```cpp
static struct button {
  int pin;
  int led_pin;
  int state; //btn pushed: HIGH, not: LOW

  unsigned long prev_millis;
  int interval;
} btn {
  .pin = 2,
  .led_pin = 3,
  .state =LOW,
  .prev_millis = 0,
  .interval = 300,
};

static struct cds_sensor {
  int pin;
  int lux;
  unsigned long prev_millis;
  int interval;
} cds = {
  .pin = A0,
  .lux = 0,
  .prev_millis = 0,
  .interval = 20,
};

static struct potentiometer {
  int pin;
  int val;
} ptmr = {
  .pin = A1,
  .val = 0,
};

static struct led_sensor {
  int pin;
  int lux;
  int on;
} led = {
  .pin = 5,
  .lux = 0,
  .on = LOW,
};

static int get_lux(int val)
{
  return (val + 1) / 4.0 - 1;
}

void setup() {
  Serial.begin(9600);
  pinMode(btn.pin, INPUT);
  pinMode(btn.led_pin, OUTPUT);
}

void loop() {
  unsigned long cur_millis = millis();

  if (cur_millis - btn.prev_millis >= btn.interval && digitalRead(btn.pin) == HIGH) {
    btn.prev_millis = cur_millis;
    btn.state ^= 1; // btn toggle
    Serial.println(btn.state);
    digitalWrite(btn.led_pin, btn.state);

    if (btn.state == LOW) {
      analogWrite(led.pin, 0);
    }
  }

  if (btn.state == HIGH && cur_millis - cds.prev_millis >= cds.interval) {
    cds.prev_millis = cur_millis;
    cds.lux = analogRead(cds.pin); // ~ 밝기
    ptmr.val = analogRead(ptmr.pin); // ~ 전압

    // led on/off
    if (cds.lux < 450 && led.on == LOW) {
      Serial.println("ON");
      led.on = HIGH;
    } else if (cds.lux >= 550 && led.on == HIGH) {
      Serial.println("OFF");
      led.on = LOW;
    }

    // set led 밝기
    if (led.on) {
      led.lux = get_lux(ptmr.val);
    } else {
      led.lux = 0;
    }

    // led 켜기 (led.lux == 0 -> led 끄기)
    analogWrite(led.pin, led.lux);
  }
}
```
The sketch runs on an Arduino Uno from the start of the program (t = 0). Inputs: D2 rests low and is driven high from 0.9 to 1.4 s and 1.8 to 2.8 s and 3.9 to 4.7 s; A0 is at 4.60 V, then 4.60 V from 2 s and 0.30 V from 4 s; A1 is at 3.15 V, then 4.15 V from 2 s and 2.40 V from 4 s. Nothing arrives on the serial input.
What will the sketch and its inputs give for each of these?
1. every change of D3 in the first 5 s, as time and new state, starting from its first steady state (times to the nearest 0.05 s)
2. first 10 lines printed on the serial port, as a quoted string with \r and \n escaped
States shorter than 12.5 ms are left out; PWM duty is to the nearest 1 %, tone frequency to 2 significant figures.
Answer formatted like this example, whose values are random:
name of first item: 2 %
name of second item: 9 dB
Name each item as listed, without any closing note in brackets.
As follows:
every change of D3 in the first 5 s, as time and new state, starting from its first steady state: 0 s low; 0.9 s high; 1.2 s low; 1.8 s high; 2.1 s low; 2.4 s high; 2.7 s low; 3.9 s high; 4.2 s low; 4.5 s high
first 10 lines printed on the serial port, as a quoted string with \r and \n escaped: "1\r\n0\r\n1\r\n0\r\n1\r\n0\r\n1\r\nON\r\n0\r\n1\r\n"
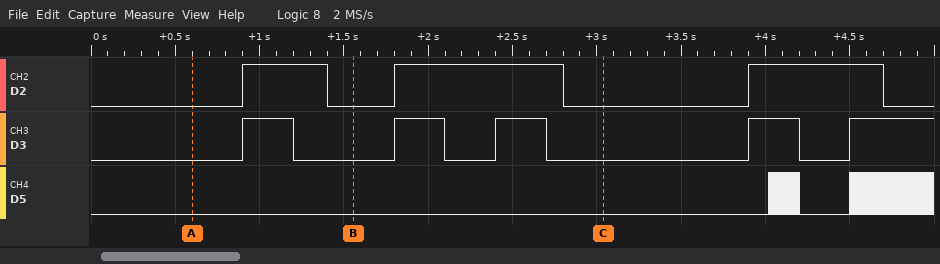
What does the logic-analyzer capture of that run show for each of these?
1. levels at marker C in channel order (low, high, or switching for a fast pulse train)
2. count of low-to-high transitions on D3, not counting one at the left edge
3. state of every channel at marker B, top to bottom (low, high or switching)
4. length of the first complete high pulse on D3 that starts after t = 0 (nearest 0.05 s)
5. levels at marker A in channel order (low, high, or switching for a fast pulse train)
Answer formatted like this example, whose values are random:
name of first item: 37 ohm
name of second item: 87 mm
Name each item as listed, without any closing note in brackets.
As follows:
levels at marker C in channel order: D2 low, D3 low, D5 low
count of low-to-high transitions on D3, not counting one at the left edge: 5
state of every channel at marker B, top to bottom: D2 low, D3 low, D5 low
length of the first complete high pulse on D3 that starts after t = 0: 0.30 s
levels at marker A in channel order: D2 low, D3 low, D5 low
